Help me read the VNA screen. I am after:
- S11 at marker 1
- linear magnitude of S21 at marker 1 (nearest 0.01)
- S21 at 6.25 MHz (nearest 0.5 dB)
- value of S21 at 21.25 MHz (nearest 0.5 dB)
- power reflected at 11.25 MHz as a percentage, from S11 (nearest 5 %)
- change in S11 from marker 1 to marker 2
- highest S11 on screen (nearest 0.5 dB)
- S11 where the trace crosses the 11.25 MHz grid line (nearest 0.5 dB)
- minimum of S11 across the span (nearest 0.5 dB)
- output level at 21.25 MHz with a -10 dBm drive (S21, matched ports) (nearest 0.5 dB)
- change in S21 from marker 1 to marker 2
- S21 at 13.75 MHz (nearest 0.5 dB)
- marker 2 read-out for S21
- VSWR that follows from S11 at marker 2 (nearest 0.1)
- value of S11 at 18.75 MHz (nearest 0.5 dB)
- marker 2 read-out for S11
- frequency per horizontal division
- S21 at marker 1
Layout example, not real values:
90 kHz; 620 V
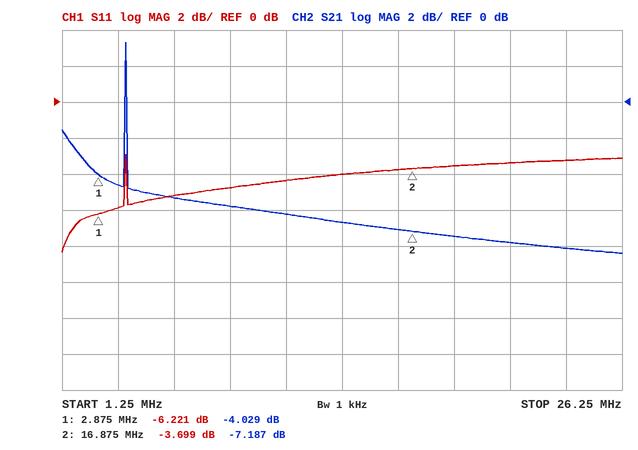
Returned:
-6.221 dB; 0.63; -5.5 dB; -8.0 dB; 35 %; 2.522 dB; -3.0 dB; -4.5 dB; -8.5 dB; -18.0 dBm; -3.158 dB; -6.5 dB; -7.187 dB; 4.8; -3.5 dB; -3.699 dB; 2.5 MHz; -4.029 dB
